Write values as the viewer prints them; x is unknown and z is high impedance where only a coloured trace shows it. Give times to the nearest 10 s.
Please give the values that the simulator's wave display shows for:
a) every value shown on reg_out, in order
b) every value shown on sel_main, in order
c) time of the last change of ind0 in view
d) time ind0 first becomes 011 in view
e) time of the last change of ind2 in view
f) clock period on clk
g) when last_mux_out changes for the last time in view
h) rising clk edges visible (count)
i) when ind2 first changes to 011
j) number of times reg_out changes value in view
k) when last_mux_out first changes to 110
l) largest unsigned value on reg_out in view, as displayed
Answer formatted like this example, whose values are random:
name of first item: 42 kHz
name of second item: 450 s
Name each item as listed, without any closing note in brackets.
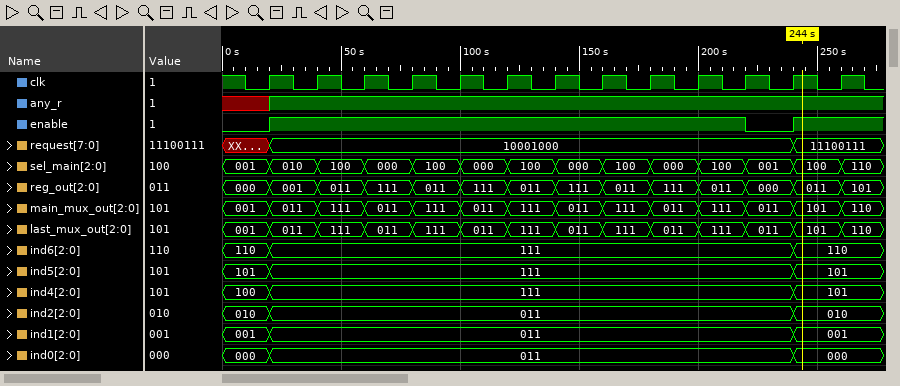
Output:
every value shown on reg_out, in order: 000, 001, 011, 111, 011, 111, 011, 111, 011, 111, 011, 000, 011, 101
every value shown on sel_main, in order: 001, 010, 100, 000, 100, 000, 100, 000, 100, 000, 100, 001, 100, 110
time of the last change of ind0 in view: 240 s
time ind0 first becomes 011 in view: 20 s
time of the last change of ind2 in view: 240 s
clock period on clk: 20 s
when last_mux_out changes for the last time in view: 260 s
rising clk edges visible: 13
when ind2 first changes to 011: 20 s
number of times reg_out changes value in view: 13
when last_mux_out first changes to 110: 260 s
largest unsigned value on reg_out in view, as displayed: 111
